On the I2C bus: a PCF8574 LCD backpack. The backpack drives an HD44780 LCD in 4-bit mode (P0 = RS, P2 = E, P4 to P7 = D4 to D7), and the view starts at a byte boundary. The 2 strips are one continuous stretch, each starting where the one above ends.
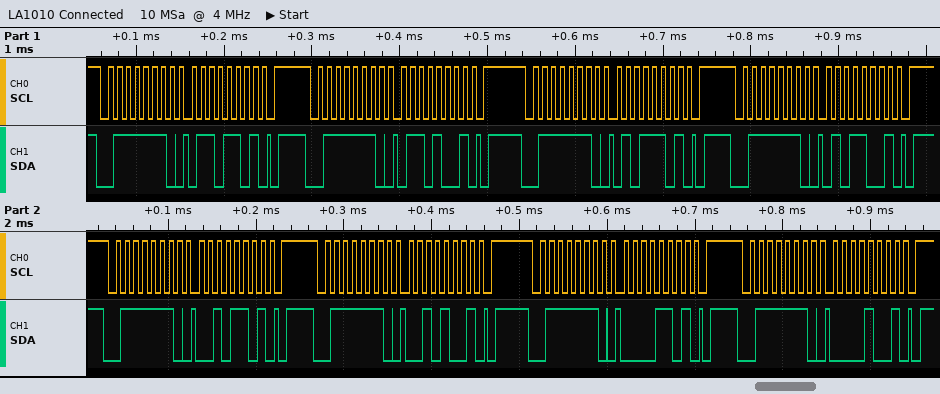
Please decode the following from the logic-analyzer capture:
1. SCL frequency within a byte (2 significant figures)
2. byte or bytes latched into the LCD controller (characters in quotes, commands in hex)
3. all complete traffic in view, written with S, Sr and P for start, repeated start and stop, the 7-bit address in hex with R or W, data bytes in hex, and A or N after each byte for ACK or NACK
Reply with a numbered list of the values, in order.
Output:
1. 100 kHz
2. 'e' ' '
3. S 3FW A 6D A P S 3FW A 69 A P S 3FW A 5D A P S 3FW A 59 A P S 3FW A 2D A P S 3FW A 29 A P S 3FW A 0D A P S 3FW A 09 A P
